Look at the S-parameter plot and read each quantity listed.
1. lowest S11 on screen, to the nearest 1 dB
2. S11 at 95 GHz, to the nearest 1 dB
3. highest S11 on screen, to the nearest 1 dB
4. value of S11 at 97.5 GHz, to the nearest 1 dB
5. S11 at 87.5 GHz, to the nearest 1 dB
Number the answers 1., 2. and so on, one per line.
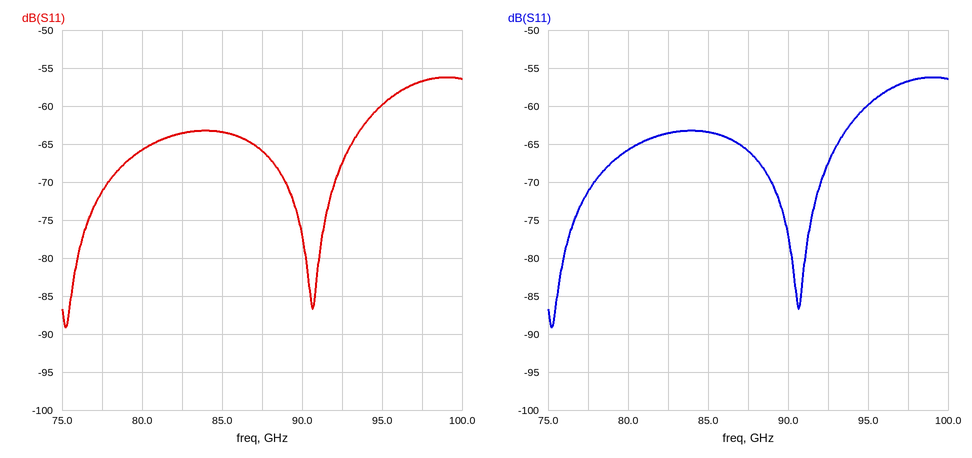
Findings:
1. -89 dB
2. -60 dB
3. -56 dB
4. -57 dB
5. -66 dB
